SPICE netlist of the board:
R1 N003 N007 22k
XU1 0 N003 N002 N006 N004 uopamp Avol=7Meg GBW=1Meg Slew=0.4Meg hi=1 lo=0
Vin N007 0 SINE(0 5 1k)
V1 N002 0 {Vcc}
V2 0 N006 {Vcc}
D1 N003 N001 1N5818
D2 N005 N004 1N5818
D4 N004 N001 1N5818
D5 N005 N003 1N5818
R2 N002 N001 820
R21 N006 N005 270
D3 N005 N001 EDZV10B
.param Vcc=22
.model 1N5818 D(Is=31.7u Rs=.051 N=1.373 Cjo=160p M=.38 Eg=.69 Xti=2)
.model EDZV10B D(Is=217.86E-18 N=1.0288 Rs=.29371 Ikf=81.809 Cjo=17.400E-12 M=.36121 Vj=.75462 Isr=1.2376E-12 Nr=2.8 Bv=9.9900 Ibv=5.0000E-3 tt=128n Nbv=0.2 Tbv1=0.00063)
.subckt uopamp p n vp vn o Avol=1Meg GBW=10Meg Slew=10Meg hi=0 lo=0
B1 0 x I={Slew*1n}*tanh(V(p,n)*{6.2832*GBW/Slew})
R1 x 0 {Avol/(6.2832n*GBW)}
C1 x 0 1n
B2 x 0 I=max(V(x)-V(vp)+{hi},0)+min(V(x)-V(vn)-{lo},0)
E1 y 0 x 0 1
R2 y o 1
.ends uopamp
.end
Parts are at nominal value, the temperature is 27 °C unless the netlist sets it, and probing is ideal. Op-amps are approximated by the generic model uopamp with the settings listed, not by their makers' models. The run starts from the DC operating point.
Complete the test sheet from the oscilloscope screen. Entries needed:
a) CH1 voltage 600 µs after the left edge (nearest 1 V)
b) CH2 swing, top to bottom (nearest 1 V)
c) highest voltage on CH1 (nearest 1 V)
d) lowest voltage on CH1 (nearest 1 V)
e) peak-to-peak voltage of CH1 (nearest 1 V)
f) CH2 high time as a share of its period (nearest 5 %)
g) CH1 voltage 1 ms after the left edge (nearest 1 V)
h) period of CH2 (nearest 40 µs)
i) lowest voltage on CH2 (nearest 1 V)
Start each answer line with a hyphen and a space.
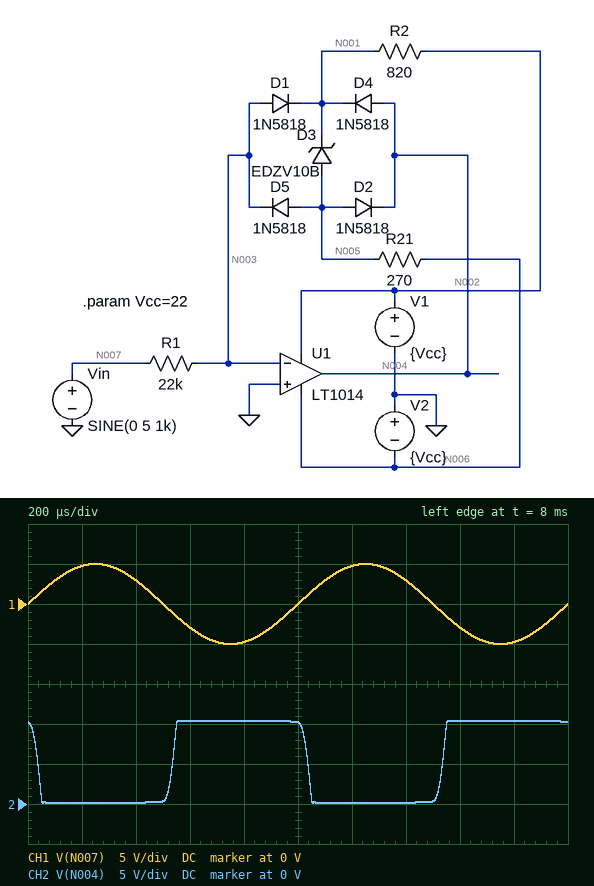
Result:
- -3 V
- 10 V
- 5 V
- -5 V
- 10 V
- 50 %
- 0 V
- 1.00 ms
- 0 V
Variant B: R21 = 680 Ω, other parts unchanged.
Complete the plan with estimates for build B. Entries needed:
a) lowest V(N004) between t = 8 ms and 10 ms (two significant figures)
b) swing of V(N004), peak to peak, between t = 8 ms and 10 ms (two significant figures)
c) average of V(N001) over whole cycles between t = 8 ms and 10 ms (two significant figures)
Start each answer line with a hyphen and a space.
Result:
- -10 V
- 21 V
- 4.9 V
